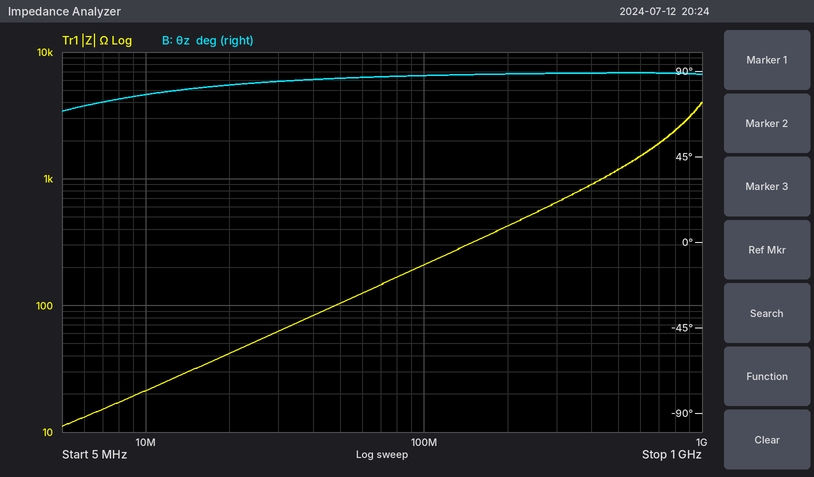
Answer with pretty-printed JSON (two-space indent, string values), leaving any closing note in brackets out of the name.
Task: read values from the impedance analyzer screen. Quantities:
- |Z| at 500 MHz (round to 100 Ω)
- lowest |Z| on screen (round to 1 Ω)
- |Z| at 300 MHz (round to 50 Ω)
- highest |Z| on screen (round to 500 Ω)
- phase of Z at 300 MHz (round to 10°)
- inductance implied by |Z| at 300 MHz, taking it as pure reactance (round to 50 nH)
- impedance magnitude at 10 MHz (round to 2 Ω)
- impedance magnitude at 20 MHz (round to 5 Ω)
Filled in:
{
  "|Z| at 500 MHz": "1.2 kΩ",
  "lowest |Z| on screen": "11 Ω",
  "|Z| at 300 MHz": "650 Ω",
  "highest |Z| on screen": "4.0 kΩ",
  "phase of Z at 300 MHz": "90°",
  "inductance implied by |Z| at 300 MHz, taking it as pure reactance": "350 nH",
  "impedance magnitude at 10 MHz": "22 Ω",
  "impedance magnitude at 20 MHz": "40 Ω"
}
